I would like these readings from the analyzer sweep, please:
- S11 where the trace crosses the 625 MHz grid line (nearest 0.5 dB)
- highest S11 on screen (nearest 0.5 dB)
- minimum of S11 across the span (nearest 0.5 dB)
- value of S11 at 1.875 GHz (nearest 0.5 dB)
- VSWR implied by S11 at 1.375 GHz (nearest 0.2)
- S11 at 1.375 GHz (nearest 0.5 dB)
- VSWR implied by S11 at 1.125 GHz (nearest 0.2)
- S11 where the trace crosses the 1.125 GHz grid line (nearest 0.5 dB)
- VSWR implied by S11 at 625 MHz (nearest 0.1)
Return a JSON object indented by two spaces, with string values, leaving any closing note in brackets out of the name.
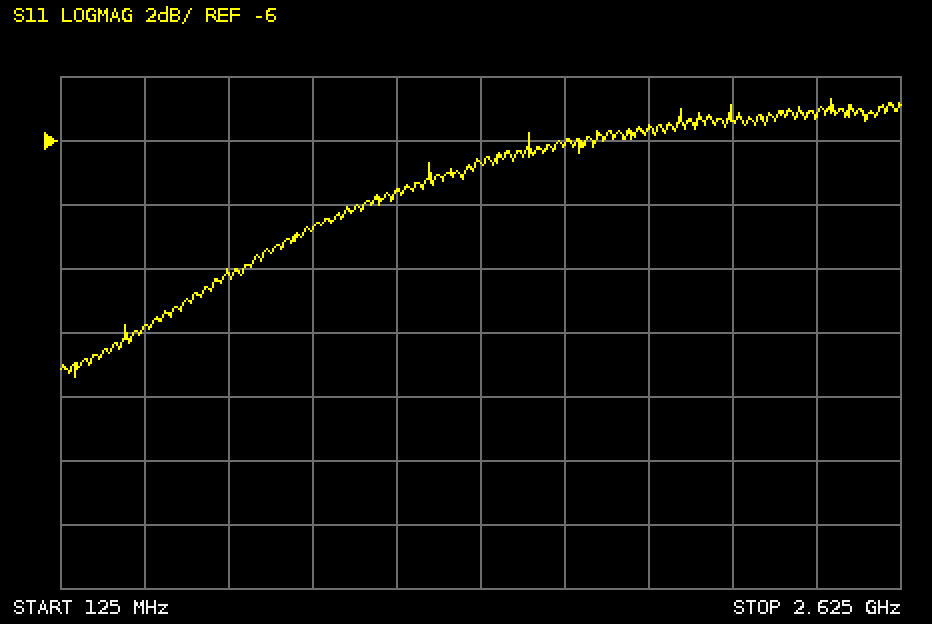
{
  "S11 where the trace crosses the 625 MHz grid line": "-10.0 dB",
  "highest S11 on screen": "-4.5 dB",
  "minimum of S11 across the span": "-13.5 dB",
  "value of S11 at 1.875 GHz": "-5.5 dB",
  "VSWR implied by S11 at 1.375 GHz": "2.8",
  "S11 at 1.375 GHz": "-6.5 dB",
  "VSWR implied by S11 at 1.125 GHz": "2.4",
  "S11 where the trace crosses the 1.125 GHz grid line": "-7.5 dB",
  "VSWR implied by S11 at 625 MHz": "1.9"
}
